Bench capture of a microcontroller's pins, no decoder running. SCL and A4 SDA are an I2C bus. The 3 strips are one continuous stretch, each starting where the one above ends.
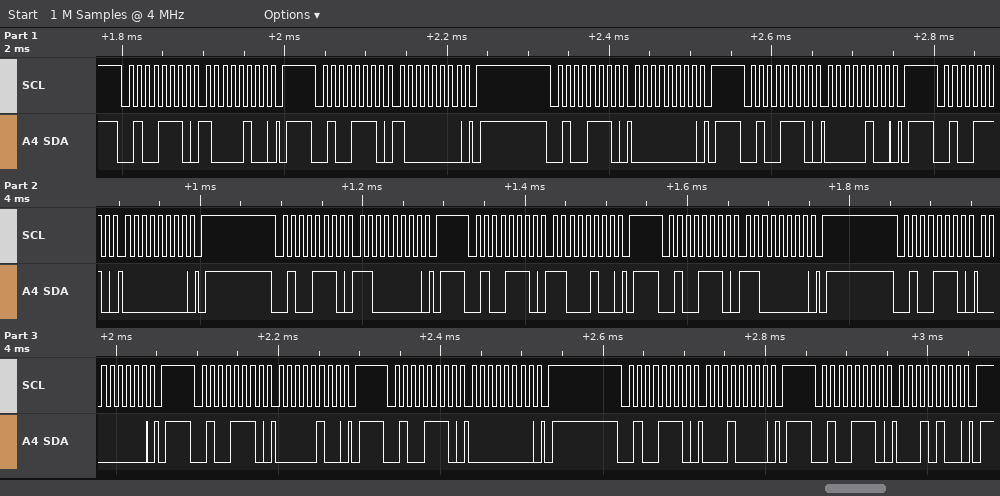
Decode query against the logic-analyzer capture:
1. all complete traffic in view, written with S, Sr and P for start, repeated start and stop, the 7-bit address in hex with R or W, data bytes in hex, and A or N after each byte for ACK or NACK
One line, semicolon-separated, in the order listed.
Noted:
S 27W A 84 A P S 27W A 80 A P S 27W A 00 A P S 27W A 04 A P S 27W A 00 A P S 27W A C0 A P S 27W A C4 A P S 27W A C0 A P S 27W A 00 A P S 27W A 04 A P S 27W A 00 A P S 27W A 10 A P S 27W A 14 A P
